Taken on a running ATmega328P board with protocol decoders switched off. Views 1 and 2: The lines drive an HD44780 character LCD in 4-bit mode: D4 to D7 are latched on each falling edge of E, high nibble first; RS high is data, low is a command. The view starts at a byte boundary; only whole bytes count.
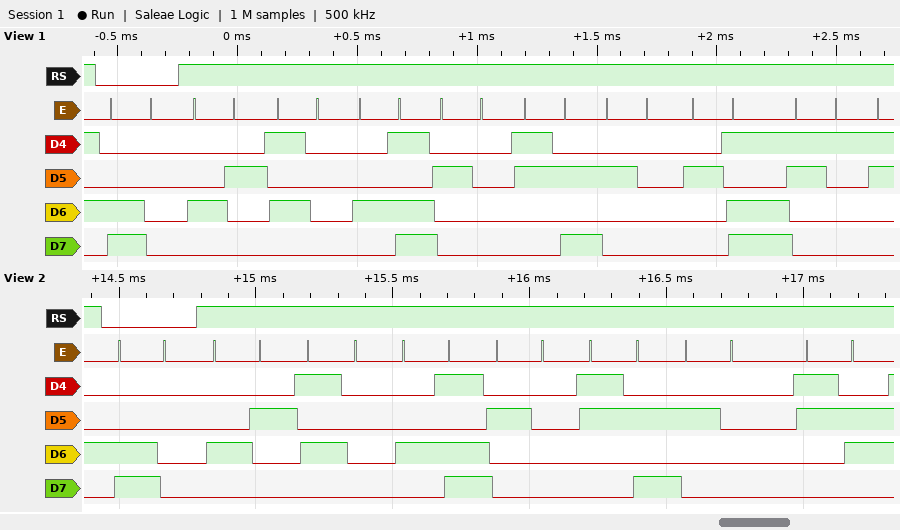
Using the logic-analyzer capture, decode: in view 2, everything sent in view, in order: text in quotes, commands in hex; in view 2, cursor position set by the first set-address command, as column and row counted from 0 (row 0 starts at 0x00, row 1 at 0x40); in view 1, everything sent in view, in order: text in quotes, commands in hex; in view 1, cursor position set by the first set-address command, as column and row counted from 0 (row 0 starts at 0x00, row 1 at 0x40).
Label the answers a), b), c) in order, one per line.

a) 0xC0 "BPM : 6"
b) column 0, row 1
c) 0xC0 "BPM : -1"
d) column 0, row 1
